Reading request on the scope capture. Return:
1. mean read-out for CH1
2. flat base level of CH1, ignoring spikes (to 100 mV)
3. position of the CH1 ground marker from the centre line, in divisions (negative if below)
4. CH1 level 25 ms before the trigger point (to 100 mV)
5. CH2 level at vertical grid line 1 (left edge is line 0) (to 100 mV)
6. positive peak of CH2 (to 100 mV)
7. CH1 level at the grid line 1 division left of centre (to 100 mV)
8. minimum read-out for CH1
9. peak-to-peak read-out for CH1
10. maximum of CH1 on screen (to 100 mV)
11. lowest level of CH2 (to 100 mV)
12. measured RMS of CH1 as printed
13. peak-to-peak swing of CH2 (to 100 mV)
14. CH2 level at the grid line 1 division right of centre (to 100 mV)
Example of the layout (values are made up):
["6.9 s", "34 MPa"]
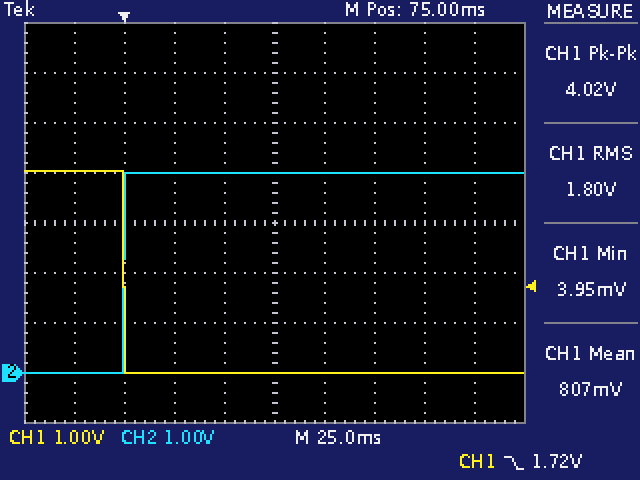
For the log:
["807 mV", "0.0 V", "-3.0 div", "4.0 V", "0.0 V", "4.0 V", "0.0 V", "3.95 mV", "4.02 V", "4.0 V", "0.0 V", "1.80 V", "4.0 V", "4.0 V"]
